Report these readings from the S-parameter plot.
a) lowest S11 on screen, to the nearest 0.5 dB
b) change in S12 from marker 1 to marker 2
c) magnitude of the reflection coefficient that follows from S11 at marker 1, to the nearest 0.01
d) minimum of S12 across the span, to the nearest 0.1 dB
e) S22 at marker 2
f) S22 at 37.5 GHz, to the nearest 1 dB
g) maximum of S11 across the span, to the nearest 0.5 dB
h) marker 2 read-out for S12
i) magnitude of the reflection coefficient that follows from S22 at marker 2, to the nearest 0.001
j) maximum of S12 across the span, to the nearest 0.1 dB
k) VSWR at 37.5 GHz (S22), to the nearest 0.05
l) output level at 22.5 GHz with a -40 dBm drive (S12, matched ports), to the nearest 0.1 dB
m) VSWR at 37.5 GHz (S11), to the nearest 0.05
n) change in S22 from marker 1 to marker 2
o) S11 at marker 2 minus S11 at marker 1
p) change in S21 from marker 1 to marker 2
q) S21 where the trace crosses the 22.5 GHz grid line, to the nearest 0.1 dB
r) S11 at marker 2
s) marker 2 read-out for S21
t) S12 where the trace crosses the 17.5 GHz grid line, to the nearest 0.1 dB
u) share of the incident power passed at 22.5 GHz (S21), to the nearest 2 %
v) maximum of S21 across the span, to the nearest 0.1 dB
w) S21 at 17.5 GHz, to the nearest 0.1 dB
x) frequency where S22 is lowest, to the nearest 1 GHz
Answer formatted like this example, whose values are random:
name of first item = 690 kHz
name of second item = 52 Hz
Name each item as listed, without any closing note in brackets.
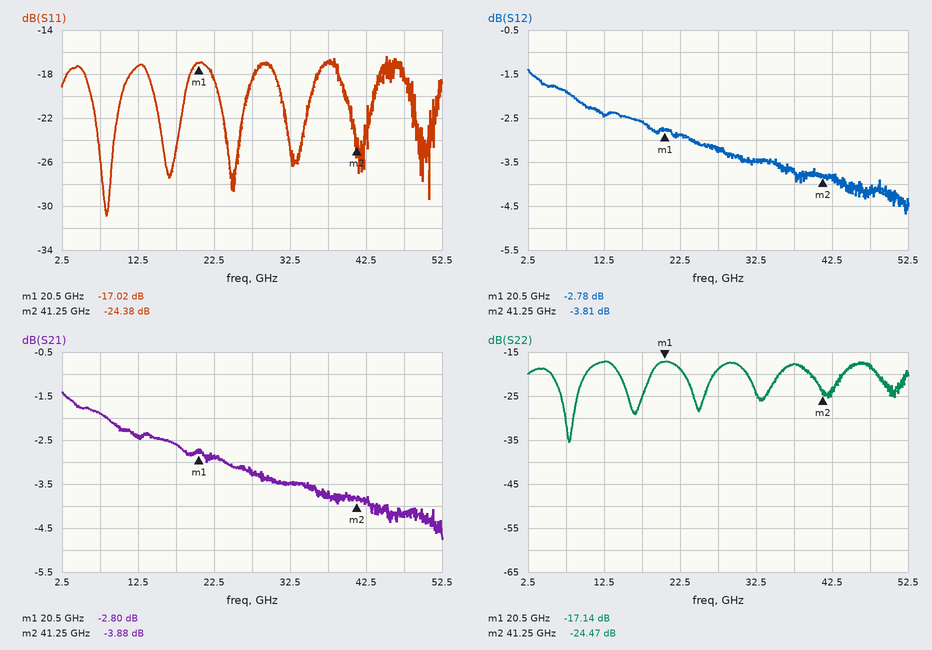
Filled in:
lowest S11 on screen, to the nearest 0.5 dB = -31.0 dB
change in S12 from marker 1 to marker 2 = -1.03 dB
magnitude of the reflection coefficient that follows from S11 at marker 1, to the nearest 0.01 = 0.14
minimum of S12 across the span, to the nearest 0.1 dB = -4.7 dB
S22 at marker 2 = -24.47 dB
S22 at 37.5 GHz, to the nearest 1 dB = -18 dB
maximum of S11 across the span, to the nearest 0.5 dB = -16.5 dB
marker 2 read-out for S12 = -3.81 dB
magnitude of the reflection coefficient that follows from S22 at marker 2, to the nearest 0.001 = 0.060
maximum of S12 across the span, to the nearest 0.1 dB = -1.4 dB
VSWR at 37.5 GHz (S22), to the nearest 0.05 = 1.30
output level at 22.5 GHz with a -40 dBm drive (S12, matched ports), to the nearest 0.1 dB = -42.9 dBm
VSWR at 37.5 GHz (S11), to the nearest 0.05 = 1.35
change in S22 from marker 1 to marker 2 = -7.33 dB
S11 at marker 2 minus S11 at marker 1 = -7.36 dB
change in S21 from marker 1 to marker 2 = -1.08 dB
S21 where the trace crosses the 22.5 GHz grid line, to the nearest 0.1 dB = -2.9 dB
S11 at marker 2 = -24.38 dB
marker 2 read-out for S21 = -3.88 dB
S12 where the trace crosses the 17.5 GHz grid line, to the nearest 0.1 dB = -2.6 dB
share of the incident power passed at 22.5 GHz (S21), to the nearest 2 % = 52 %
maximum of S21 across the span, to the nearest 0.1 dB = -1.4 dB
S21 at 17.5 GHz, to the nearest 0.1 dB = -2.6 dB
frequency where S22 is lowest, to the nearest 1 GHz = 8 GHz
